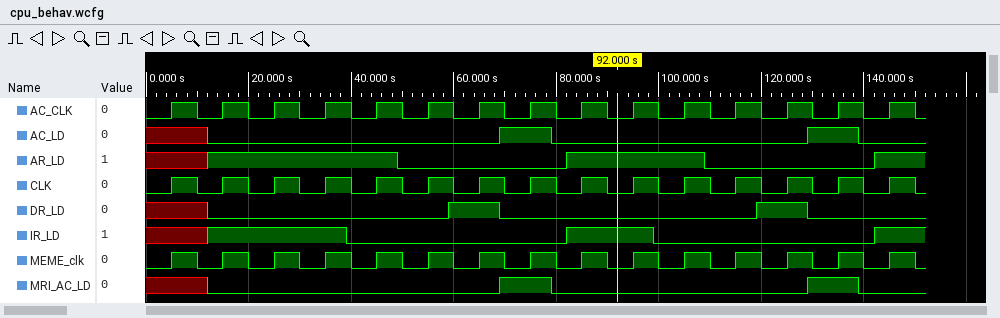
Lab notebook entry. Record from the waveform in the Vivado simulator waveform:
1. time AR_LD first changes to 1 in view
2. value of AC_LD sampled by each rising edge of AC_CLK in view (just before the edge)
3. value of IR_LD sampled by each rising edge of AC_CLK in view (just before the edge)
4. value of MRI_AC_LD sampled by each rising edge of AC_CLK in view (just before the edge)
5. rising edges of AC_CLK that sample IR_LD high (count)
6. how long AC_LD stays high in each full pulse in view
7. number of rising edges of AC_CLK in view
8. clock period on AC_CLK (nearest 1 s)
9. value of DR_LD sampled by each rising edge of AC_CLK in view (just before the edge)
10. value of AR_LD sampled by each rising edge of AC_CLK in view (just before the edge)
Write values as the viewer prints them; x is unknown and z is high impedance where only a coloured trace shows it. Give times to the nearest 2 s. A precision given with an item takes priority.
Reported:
12 s
x 0 0 0 0 0 0 1 0 0 0 0 0 1 0
x 1 1 1 0 0 0 0 1 1 0 0 0 0 1
x 0 0 0 0 0 0 1 0 0 0 0 0 1 0
6
10 s, 10 s
15
10 s
x 0 0 0 0 0 1 0 0 0 0 0 1 0 0
x 1 1 1 1 0 0 0 1 1 1 0 0 0 1
